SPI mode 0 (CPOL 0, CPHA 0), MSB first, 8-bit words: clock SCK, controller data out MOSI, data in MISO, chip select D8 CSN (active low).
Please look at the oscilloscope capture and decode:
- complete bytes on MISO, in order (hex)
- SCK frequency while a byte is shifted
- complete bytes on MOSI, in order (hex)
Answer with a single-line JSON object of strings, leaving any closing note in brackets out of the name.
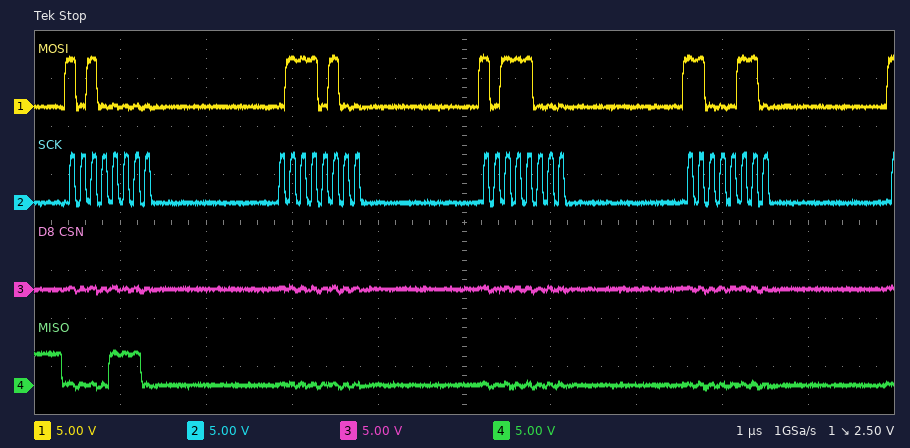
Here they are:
{"complete bytes on MISO, in order": "0E 00 00 00", "SCK frequency while a byte is shifted": "8 MHz", "complete bytes on MOSI, in order": "A0 74 B8 C6"}
